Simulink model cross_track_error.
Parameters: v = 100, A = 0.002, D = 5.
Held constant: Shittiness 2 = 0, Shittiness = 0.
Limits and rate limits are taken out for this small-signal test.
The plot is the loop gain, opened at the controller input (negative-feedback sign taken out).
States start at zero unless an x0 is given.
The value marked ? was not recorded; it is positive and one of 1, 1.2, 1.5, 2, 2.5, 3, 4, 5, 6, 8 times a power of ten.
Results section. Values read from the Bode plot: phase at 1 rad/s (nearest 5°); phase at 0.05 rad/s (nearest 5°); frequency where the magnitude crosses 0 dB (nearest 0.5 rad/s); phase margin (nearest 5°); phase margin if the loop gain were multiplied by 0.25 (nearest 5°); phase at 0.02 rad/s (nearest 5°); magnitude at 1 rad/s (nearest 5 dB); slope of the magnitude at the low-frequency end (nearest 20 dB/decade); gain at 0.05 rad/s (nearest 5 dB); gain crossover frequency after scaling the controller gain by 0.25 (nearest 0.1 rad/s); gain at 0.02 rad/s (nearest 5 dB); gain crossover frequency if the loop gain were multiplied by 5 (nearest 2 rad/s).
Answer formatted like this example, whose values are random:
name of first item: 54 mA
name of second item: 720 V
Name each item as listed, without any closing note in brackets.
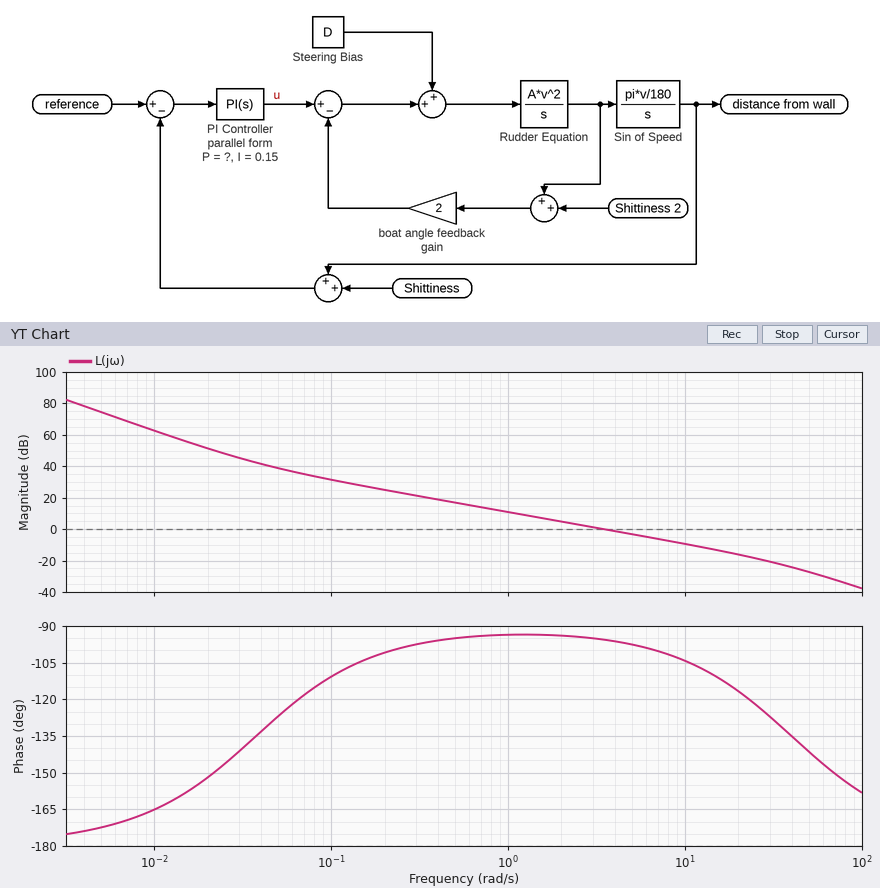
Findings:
phase at 1 rad/s: -95°
phase at 0.05 rad/s: -125°
frequency where the magnitude crosses 0 dB: 3.5 rad/s
phase margin: 85°
phase margin if the loop gain were multiplied by 0.25: 85°
phase at 0.02 rad/s: -150°
magnitude at 1 rad/s: 10 dB
slope of the magnitude at the low-frequency end: -40 dB/decade
gain at 0.05 rad/s: 40 dB
gain crossover frequency after scaling the controller gain by 0.25: 0.9 rad/s
gain at 0.02 rad/s: 50 dB
gain crossover frequency if the loop gain were multiplied by 5: 16 rad/s
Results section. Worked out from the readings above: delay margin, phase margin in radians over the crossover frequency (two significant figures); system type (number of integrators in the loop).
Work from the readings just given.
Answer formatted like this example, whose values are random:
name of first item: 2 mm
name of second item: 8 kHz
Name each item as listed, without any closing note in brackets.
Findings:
delay margin, phase margin in radians over the crossover frequency: 0.42 s
system type: 2
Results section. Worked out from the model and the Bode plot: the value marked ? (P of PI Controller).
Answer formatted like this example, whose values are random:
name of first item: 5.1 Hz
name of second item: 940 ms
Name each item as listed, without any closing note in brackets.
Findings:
the value marked ?: 4
